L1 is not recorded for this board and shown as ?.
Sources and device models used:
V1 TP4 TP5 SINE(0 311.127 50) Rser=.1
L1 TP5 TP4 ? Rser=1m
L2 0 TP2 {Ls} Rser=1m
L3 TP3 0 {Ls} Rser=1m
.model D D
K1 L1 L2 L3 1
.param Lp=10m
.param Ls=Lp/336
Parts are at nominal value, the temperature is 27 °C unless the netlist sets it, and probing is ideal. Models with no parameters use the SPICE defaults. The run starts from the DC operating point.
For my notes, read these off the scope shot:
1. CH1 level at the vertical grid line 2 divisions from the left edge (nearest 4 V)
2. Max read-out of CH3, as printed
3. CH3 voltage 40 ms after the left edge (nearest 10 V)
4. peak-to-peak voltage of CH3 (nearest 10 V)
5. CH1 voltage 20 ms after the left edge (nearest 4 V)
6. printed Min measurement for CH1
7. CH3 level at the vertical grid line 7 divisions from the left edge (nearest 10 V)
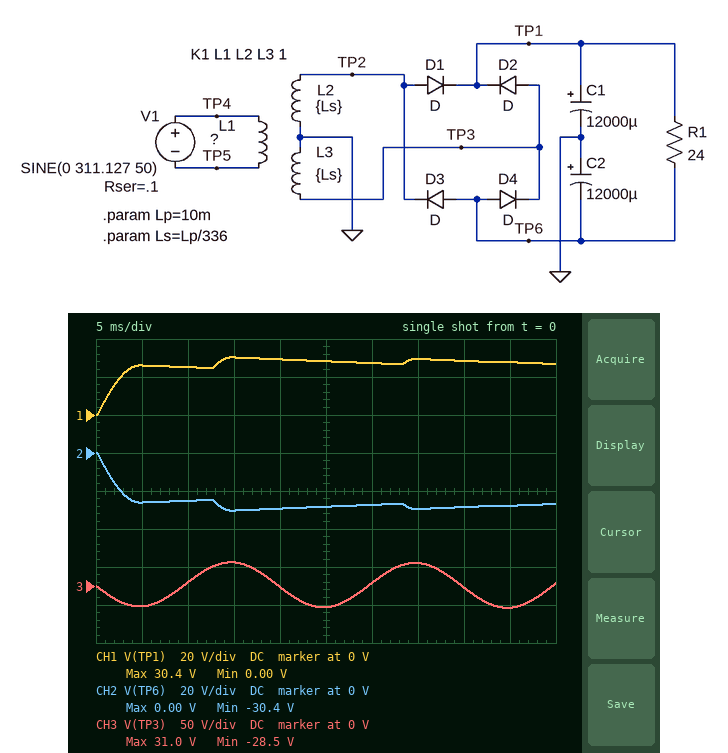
24 V
31.0 V
0 V
60 V
28 V
0.00 V
30 V
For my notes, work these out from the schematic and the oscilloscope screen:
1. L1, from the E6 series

3.3 mH
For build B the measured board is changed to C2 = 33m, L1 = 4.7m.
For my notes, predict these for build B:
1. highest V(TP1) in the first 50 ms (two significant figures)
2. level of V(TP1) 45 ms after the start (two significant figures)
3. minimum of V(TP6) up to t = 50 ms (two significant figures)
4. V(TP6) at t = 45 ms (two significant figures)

25 V
23 V
-25 V
-24 V
